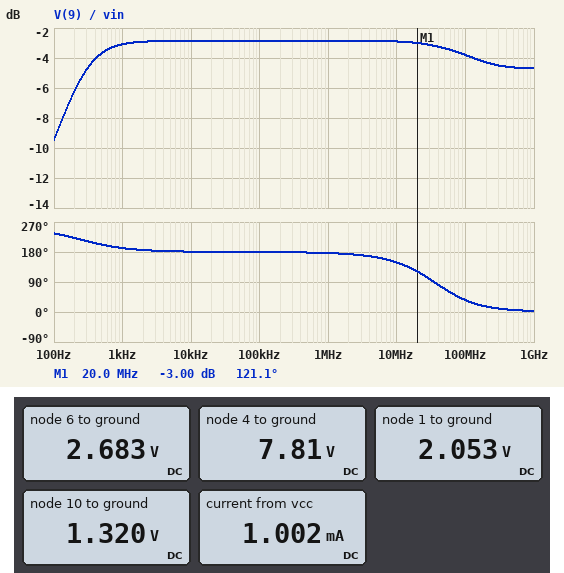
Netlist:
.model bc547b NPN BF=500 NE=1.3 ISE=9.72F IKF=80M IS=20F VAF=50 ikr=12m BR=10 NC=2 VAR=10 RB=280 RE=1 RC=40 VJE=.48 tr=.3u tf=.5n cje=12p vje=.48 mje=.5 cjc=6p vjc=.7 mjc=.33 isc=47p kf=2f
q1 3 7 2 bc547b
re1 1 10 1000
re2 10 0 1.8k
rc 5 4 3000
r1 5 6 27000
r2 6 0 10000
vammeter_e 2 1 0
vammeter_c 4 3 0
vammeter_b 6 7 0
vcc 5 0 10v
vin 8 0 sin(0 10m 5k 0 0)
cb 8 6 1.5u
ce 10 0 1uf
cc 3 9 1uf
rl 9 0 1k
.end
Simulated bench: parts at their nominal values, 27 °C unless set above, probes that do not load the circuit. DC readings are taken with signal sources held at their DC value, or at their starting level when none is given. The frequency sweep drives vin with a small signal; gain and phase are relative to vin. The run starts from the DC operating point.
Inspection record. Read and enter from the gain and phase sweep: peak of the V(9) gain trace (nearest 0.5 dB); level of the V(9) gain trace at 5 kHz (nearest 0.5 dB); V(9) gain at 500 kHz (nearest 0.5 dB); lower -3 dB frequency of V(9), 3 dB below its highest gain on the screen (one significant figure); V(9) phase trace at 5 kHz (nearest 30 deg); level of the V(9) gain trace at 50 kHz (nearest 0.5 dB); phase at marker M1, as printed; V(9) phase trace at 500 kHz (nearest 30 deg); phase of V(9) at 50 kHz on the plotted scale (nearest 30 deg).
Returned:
-3.0 dB
-3.0 dB
-3.0 dB
200 Hz
180 deg
-3.0 dB
121.1 deg
180 deg
180 deg
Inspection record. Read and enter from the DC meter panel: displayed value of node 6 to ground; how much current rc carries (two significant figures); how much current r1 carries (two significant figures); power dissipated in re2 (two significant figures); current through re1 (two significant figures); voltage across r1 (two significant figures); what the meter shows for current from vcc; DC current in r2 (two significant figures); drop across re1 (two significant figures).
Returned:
2.683 V
730 µA
270 µA
970 µW
730 µA
7.3 V
1.002 mA
270 µA
730 mV
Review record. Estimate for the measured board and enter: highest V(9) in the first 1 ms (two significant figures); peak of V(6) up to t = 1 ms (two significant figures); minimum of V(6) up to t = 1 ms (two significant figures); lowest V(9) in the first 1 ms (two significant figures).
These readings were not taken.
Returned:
7.4 mV
2.7 V
2.7 V
-7.1 mV
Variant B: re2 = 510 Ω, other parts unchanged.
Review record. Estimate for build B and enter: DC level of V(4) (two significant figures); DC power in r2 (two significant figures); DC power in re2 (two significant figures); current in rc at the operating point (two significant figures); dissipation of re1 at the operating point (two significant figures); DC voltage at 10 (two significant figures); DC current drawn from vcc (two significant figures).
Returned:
6.0 V
710 µW
910 µW
1.3 mA
1.8 mW
680 mV
1.6 mA
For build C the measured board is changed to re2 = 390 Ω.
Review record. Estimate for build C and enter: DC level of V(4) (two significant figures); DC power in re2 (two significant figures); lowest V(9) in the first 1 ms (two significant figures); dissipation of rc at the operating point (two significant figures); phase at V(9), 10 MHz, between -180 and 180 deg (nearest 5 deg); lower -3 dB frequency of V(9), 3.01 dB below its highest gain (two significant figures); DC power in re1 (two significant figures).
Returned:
5.7 V
820 µW
-7.2 mV
6.3 mW
145 deg
140 Hz
2.1 mW
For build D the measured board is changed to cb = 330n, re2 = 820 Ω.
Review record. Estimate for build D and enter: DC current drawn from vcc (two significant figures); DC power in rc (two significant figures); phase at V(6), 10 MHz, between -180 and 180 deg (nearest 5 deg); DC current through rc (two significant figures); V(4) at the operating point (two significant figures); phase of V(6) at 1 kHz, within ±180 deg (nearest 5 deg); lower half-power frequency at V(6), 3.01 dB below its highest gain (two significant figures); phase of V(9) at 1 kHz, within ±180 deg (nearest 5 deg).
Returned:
1.4 mA
3.7 mW
0 deg
1.1 mA
6.7 V
5 deg
67 Hz
-165 deg
